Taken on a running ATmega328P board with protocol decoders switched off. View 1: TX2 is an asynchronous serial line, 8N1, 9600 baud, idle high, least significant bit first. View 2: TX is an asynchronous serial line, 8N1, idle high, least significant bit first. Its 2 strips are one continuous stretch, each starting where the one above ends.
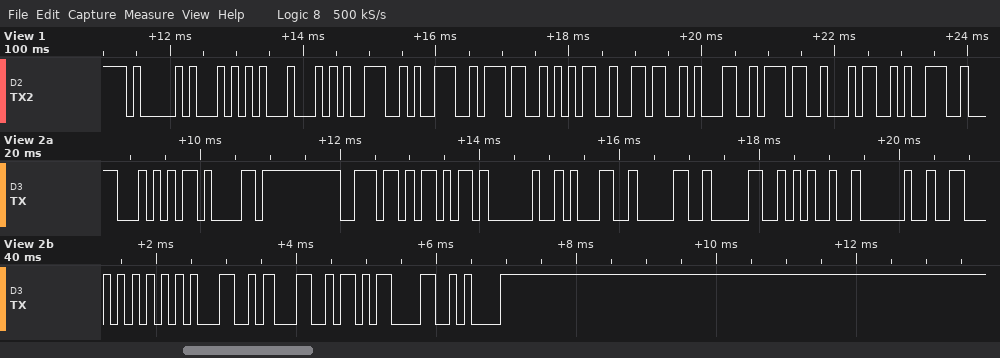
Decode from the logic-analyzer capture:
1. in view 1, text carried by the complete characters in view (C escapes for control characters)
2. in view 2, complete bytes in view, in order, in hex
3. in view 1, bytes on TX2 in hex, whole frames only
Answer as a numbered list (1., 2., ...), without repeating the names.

1. "ATD997561749"
2. 54 61 6E 6B 20 31 30 30 25 20 46 55 4C 4C 0D 0A
3. 41 54 44 39 39 37 35 36 31 37 34 39
